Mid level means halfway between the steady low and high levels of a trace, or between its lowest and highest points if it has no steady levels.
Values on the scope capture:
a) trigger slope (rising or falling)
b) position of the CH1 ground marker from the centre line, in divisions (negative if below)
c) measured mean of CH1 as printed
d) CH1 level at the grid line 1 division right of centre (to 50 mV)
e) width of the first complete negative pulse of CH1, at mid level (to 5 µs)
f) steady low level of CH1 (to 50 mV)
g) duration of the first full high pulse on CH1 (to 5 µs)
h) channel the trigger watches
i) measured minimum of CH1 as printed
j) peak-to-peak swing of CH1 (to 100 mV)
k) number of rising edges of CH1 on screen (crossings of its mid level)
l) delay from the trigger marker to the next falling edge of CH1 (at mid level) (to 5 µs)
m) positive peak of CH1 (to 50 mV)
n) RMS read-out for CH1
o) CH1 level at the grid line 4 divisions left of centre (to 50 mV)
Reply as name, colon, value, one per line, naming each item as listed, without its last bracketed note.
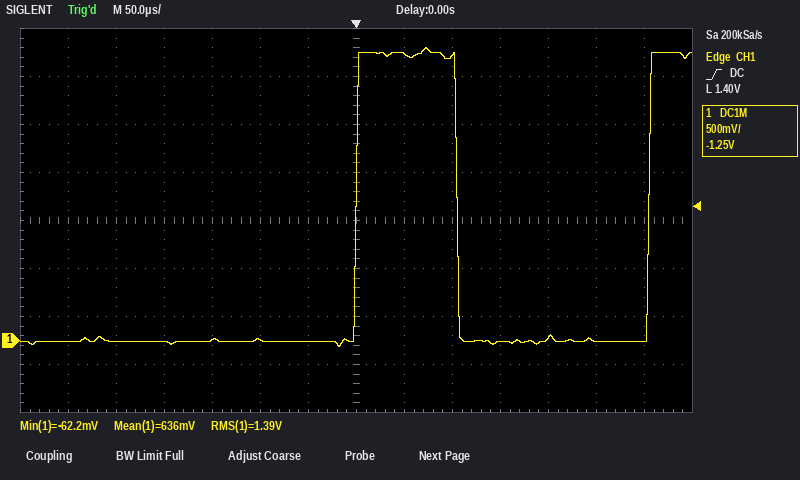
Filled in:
trigger slope: rising
position of the CH1 ground marker from the centre line, in divisions: -2.5 div
measured mean of CH1 as printed: 636 mV
CH1 level at the grid line 1 division right of centre: 3.00 V
width of the first complete negative pulse of CH1, at mid level: 200 µs
steady low level of CH1: 0 mV
duration of the first full high pulse on CH1: 105 µs
channel the trigger watches: CH1
measured minimum of CH1 as printed: -62.2 mV
peak-to-peak swing of CH1: 3.10 V
number of rising edges of CH1 on screen: 2
delay from the trigger marker to the next falling edge of CH1 (at mid level): 105 µs
positive peak of CH1: 3.05 V
RMS read-out for CH1: 1.39 V
CH1 level at the grid line 4 divisions left of centre: 0 mV
